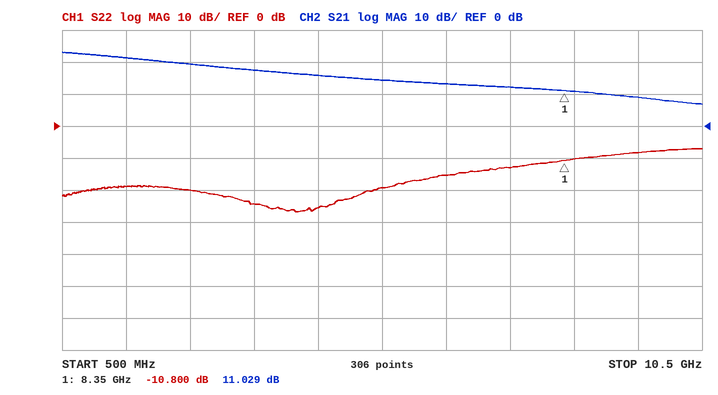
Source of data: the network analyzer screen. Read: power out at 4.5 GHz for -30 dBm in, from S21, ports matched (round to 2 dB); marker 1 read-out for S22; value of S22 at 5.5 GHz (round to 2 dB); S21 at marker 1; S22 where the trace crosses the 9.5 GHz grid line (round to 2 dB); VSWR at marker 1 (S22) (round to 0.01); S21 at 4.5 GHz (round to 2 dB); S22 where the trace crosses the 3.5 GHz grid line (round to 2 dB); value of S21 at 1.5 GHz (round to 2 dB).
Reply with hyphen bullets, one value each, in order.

- -14 dBm
- -10.800 dB
- -20 dB
- 11.029 dB
- -8 dB
- 1.81
- 16 dB
- -24 dB
- 22 dB
